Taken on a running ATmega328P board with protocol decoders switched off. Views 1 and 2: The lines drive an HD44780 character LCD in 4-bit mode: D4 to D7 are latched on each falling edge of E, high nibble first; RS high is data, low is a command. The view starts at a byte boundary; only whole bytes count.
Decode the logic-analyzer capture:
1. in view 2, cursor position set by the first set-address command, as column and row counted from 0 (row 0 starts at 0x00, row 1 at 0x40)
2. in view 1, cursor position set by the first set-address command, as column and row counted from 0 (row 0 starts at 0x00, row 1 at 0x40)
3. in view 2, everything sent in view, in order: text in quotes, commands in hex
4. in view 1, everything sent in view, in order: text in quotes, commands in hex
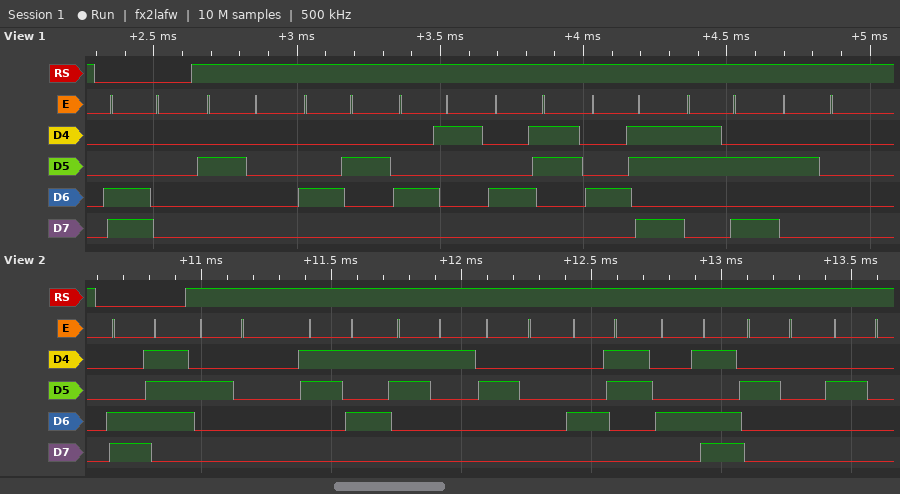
column 7, row 1
column 0, row 1
0xC7 " 51 CM  "
0xC0 " BACK: "
